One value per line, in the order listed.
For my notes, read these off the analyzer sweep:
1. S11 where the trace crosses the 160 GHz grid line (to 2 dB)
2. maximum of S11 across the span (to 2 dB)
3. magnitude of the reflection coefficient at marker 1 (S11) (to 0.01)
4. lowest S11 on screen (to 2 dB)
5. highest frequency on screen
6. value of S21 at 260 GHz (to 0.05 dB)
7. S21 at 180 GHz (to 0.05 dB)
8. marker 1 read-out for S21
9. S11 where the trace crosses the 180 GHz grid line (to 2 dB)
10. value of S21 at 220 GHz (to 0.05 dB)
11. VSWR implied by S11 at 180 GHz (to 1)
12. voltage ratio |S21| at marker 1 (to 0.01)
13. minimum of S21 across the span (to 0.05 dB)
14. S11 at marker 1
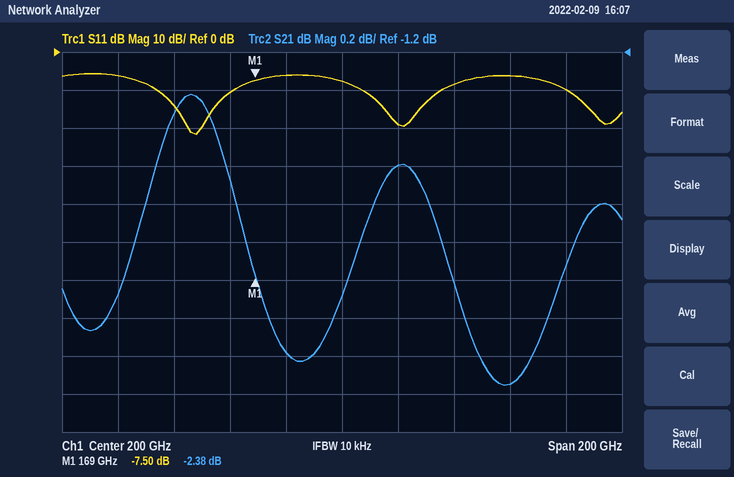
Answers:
-10 dB
-6 dB
0.42
-22 dB
300 GHz
-2.95 dB
-2.80 dB
-2.38 dB
-6 dB
-1.80 dB
3
0.76
-2.95 dB
-7.50 dB
